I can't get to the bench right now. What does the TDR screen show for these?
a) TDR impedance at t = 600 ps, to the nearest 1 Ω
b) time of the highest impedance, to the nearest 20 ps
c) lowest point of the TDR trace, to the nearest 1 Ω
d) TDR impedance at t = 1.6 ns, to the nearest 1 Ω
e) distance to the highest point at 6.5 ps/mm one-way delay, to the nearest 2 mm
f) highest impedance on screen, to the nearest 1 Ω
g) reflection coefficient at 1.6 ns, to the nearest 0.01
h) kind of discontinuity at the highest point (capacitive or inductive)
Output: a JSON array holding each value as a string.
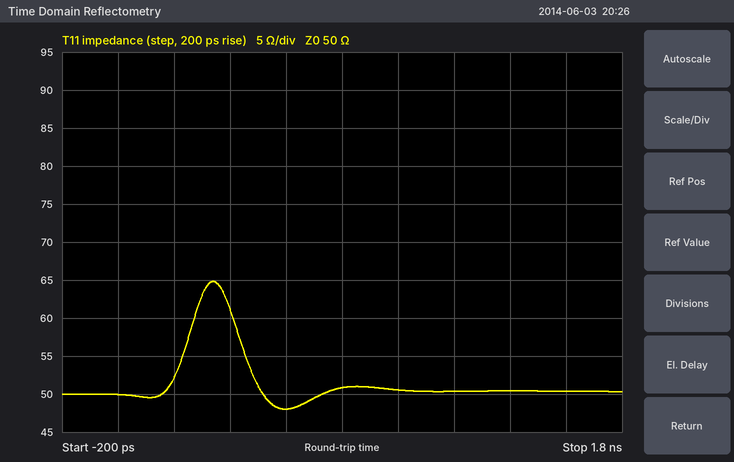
["48 Ω", "340 ps", "48 Ω", "50 Ω", "26 mm", "65 Ω", "0.00", "inductive"]
